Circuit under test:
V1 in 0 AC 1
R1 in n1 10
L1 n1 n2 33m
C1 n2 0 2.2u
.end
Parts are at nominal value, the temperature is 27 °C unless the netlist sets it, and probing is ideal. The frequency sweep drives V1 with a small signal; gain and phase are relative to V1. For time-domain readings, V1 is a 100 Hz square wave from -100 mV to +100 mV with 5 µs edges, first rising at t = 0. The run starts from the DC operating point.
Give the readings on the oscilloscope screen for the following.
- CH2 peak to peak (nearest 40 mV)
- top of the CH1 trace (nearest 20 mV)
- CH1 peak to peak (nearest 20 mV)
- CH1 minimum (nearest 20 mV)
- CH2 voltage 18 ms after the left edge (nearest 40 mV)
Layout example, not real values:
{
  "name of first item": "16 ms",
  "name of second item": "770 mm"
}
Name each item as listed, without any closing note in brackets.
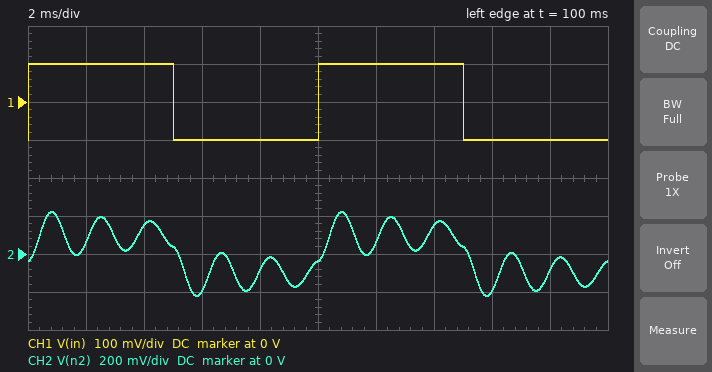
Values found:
{
  "CH2 peak to peak": "440 mV",
  "top of the CH1 trace": "100 mV",
  "CH1 peak to peak": "200 mV",
  "CH1 minimum": "-100 mV",
  "CH2 voltage 18 ms after the left edge": "-80 mV"
}
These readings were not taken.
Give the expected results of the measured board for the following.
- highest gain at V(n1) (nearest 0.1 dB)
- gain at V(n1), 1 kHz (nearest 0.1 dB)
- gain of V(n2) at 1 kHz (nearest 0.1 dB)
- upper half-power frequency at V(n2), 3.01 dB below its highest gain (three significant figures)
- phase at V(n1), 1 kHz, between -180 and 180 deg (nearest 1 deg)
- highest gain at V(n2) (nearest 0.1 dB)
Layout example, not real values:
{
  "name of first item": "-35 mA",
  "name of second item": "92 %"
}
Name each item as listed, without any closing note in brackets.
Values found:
{
  "highest gain at V(n1)": "0 dB",
  "gain at V(n1), 1 kHz": "0 dB",
  "gain of V(n2) at 1 kHz": "-5.4 dB",
  "upper half-power frequency at V(n2), 3.01 dB below its highest gain": "613 Hz",
  "phase at V(n1), 1 kHz, between -180 and 180 deg": "4 deg",
  "highest gain at V(n2)": "21.8 dB"
}
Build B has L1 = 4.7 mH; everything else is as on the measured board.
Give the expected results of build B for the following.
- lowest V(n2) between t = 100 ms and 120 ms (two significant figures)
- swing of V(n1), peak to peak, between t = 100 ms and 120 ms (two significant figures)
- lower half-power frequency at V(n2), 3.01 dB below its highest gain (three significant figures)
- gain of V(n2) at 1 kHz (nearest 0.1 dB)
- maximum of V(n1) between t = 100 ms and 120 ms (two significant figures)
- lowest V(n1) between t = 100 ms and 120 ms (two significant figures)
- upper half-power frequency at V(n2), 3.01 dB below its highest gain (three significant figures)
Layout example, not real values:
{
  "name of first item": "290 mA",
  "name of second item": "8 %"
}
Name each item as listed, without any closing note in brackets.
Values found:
{
  "lowest V(n2) between t = 100 ms and 120 ms": "-240 mV",
  "swing of V(n1), peak to peak, between t = 100 ms and 120 ms": "250 mV",
  "lower half-power frequency at V(n2), 3.01 dB below its highest gain": "1.37 kHz",
  "gain of V(n2) at 1 kHz": "4.3 dB",
  "maximum of V(n1) between t = 100 ms and 120 ms": "130 mV",
  "lowest V(n1) between t = 100 ms and 120 ms": "-130 mV",
  "upper half-power frequency at V(n2), 3.01 dB below its highest gain": "1.71 kHz"
}
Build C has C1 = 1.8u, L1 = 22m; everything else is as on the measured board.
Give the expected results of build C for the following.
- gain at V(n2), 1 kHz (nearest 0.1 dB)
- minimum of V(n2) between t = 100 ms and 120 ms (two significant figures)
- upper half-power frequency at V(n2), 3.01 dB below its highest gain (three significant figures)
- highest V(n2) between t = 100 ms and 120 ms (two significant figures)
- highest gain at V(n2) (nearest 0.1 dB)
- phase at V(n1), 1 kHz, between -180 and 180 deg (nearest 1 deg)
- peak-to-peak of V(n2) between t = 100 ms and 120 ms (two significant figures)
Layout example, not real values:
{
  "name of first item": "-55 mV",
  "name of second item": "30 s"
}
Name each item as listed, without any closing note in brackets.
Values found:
{
  "gain at V(n2), 1 kHz": "4.8 dB",
  "minimum of V(n2) between t = 100 ms and 120 ms": "-230 mV",
  "upper half-power frequency at V(n2), 3.01 dB below its highest gain": "834 Hz",
  "highest V(n2) between t = 100 ms and 120 ms": "230 mV",
  "highest gain at V(n2)": "20.9 dB",
  "phase at V(n1), 1 kHz, between -180 and 180 deg": "11 deg",
  "peak-to-peak of V(n2) between t = 100 ms and 120 ms": "460 mV"
}
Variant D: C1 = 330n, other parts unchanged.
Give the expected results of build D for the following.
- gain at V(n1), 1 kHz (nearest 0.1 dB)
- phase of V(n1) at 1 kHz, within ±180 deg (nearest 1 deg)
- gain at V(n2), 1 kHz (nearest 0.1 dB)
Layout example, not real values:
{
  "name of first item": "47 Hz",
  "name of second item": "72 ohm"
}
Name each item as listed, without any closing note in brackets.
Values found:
{
  "gain at V(n1), 1 kHz": "0 dB",
  "phase of V(n1) at 1 kHz, within ±180 deg": "-2 deg",
  "gain at V(n2), 1 kHz": "4.9 dB"
}
